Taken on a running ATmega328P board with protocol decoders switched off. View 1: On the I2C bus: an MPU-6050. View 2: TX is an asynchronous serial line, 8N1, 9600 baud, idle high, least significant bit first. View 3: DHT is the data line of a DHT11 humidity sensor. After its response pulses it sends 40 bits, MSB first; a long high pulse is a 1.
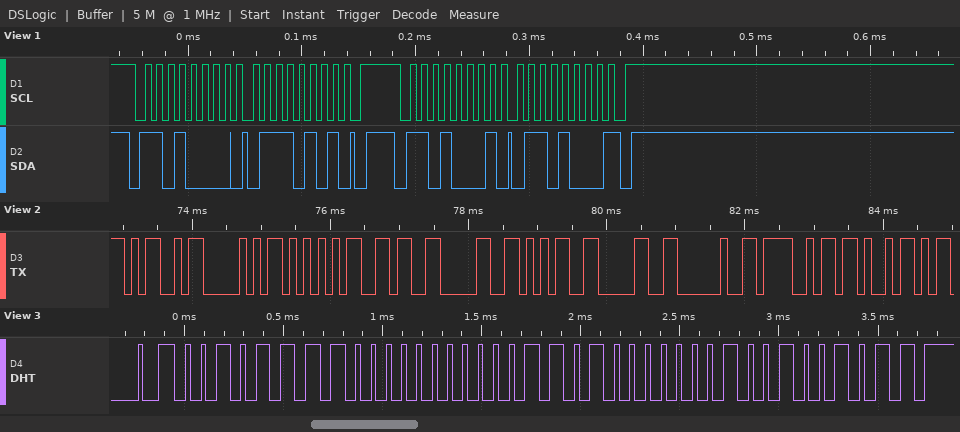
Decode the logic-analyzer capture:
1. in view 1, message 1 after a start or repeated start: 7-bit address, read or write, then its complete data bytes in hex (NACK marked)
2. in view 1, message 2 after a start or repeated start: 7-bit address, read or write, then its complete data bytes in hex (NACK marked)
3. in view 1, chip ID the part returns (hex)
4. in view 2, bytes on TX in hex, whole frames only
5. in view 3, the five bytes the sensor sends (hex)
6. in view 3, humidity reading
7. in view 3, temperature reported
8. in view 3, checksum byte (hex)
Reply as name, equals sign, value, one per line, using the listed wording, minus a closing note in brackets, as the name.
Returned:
in view 1, message 1 after a start or repeated start: 7-bit address, read or write, then its complete data bytes in hex = 0x68 write: 75
in view 1, message 2 after a start or repeated start: 7-bit address, read or write, then its complete data bytes in hex = 0x68 read: 68 NACK
in view 1, chip ID the part returns = 0x68
in view 2, bytes on TX in hex, whole frames only = 4D 50 55 36 30 35 30 20 4F 4B
in view 3, the five bytes the sensor sends = 2F 00 1A 02 4B
in view 3, humidity reading = 47 %
in view 3, temperature reported = 26.2 °C
in view 3, checksum byte = 0x4B
